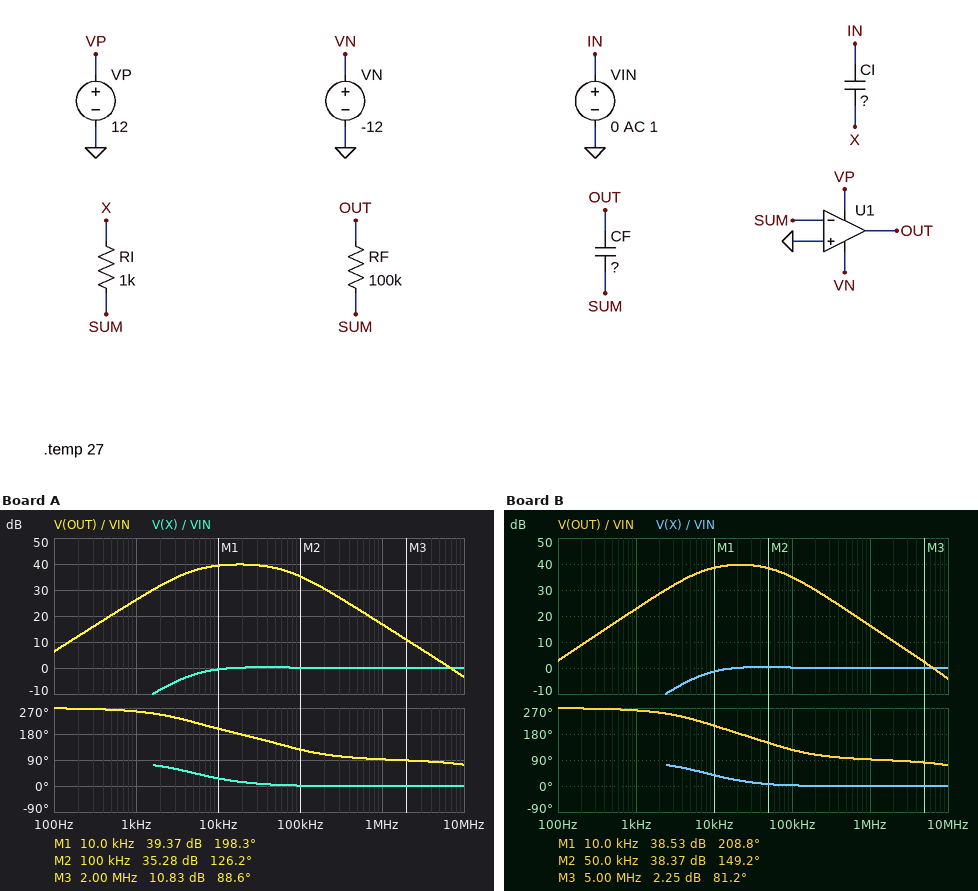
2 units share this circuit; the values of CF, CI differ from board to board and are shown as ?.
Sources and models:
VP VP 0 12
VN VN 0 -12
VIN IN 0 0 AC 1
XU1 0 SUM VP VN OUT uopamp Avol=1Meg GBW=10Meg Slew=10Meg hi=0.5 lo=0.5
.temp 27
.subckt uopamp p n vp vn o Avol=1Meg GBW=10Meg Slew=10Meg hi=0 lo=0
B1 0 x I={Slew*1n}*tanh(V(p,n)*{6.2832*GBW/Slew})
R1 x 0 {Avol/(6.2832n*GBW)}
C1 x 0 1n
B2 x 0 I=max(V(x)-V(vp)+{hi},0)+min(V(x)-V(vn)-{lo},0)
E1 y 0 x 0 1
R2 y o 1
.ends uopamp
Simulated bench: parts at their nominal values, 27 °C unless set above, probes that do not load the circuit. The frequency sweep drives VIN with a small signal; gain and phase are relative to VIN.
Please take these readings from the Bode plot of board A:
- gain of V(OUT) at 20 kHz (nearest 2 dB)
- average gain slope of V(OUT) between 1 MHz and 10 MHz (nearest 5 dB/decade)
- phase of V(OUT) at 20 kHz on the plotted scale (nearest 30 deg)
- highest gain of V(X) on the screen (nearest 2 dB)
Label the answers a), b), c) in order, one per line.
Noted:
a) 40 dB
b) -20 dB/decade
c) 180 deg
d) 0 dB
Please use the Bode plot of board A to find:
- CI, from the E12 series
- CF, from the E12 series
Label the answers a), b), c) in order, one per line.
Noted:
a) 33 nF
b) 6.8 pF
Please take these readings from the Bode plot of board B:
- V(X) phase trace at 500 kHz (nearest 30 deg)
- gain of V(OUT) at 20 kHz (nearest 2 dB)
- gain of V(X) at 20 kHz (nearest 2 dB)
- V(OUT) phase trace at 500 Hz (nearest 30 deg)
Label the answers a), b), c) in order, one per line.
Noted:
a) 0 deg
b) 40 dB
c) 0 dB
d) 270 deg
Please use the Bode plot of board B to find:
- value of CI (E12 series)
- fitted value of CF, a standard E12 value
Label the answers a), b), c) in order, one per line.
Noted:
a) 22 nF
b) 8.2 pF
